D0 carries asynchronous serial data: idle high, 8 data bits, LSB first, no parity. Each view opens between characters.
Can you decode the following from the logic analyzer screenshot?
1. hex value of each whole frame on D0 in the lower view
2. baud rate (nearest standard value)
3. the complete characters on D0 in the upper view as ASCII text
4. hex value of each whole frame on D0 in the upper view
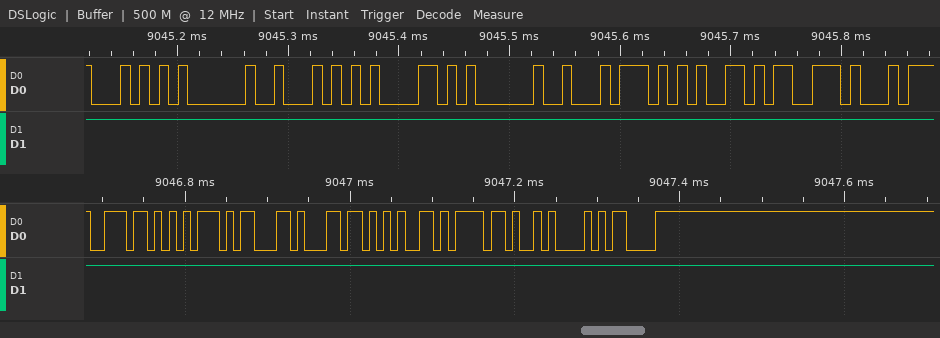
6E, 75, 63, 6C, 65, 6F, 0A, 0D
115200 baud
"T TX tes"
54, 20, 54, 58, 20, 74, 65, 73
